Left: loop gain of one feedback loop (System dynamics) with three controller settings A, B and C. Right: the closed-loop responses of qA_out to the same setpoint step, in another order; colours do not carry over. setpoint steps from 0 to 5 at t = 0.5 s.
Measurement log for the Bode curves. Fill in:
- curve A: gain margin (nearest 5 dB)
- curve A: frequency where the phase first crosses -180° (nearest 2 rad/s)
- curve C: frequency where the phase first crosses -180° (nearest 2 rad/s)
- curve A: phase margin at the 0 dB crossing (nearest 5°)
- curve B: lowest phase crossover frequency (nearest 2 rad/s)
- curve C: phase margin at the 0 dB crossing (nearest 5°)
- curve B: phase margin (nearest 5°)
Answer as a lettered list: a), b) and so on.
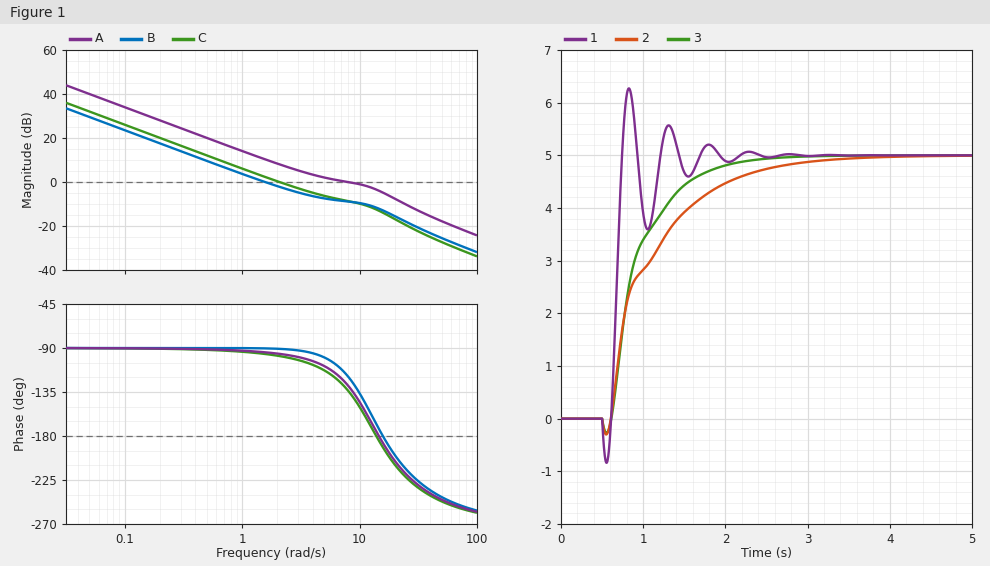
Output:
a) 5 dB
b) 14 rad/s
c) 14 rad/s
d) 50°
e) 16 rad/s
f) 80°
g) 90°
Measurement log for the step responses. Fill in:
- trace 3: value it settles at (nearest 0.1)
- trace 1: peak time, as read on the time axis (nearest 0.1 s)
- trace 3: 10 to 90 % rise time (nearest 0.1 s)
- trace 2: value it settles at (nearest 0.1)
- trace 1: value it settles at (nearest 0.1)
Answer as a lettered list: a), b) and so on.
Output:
a) 5.0
b) 0.8 s
c) 0.9 s
d) 5.0
e) 5.0
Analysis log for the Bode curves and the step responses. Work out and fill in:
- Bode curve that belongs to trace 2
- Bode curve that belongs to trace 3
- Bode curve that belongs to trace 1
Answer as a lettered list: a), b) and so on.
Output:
a) B
b) C
c) A
